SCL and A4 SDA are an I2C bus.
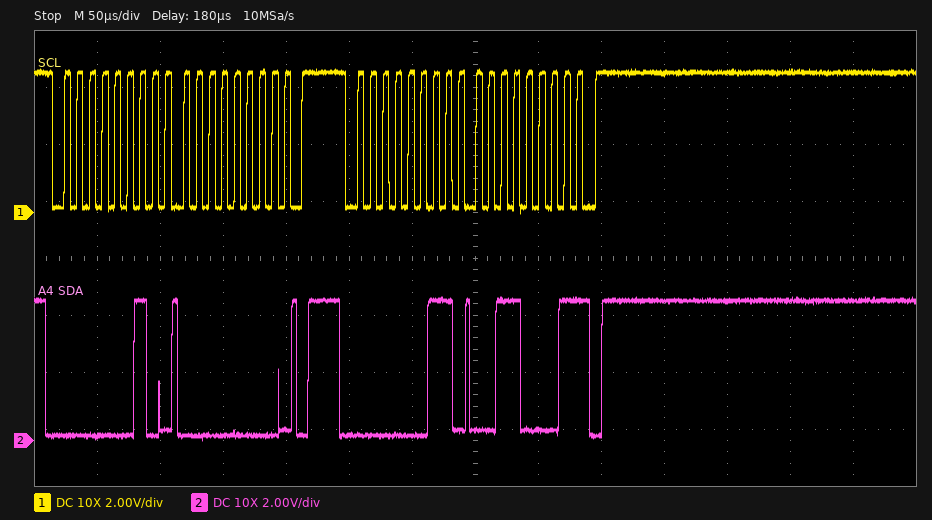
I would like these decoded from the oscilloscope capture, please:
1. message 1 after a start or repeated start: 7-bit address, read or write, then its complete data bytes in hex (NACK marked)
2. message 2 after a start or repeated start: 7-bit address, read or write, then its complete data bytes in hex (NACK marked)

0x01 write: 00
0x01 read: 31 NACK
